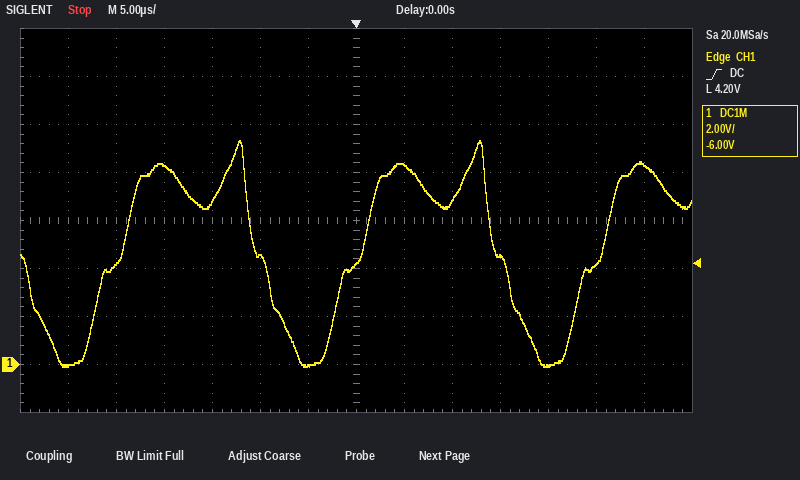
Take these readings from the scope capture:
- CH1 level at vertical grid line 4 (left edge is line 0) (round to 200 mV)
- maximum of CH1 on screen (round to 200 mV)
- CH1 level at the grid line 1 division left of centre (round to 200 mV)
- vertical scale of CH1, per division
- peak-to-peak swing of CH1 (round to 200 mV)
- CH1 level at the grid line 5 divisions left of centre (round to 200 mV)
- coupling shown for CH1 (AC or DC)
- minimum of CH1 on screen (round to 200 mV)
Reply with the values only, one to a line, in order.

6.8 V
9.4 V
0.0 V
2 V
9.4 V
4.2 V
DC
0.0 V
